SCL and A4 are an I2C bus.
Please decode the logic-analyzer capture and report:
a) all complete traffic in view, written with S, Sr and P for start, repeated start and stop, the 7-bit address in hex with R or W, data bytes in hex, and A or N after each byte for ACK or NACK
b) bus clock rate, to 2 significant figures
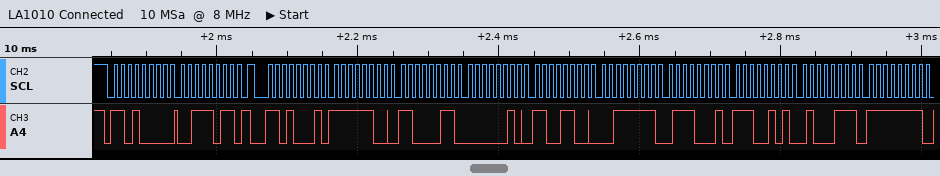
S 68W A 3B A Sr 68R A FC A C3 A 02 A CC A 3F A 71 A E5 A 47 A FF A
100 kHz
